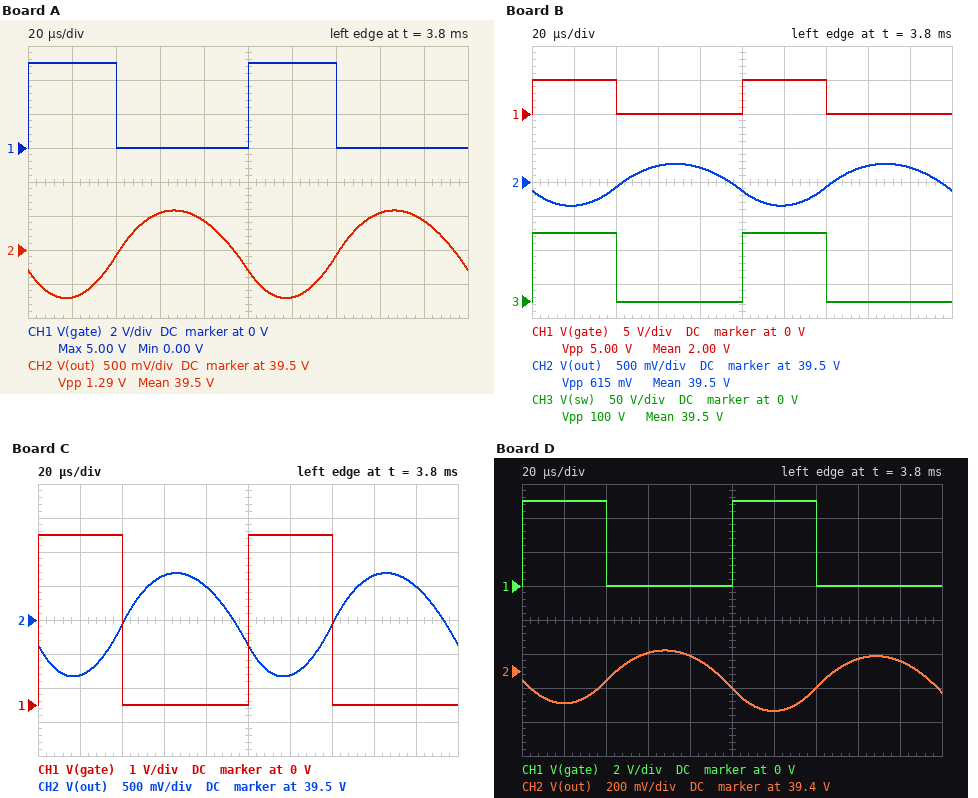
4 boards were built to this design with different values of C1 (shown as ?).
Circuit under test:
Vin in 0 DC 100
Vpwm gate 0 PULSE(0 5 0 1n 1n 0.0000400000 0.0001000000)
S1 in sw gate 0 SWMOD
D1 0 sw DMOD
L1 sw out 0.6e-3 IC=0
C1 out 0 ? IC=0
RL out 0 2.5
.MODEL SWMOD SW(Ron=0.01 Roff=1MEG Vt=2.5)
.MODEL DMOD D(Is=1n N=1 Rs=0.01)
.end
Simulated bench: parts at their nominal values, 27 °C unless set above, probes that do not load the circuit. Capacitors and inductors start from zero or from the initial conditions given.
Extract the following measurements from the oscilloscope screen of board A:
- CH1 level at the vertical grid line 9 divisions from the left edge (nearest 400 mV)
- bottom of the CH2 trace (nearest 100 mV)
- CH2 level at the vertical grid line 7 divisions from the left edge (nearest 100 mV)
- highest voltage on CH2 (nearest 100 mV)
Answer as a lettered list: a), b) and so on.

a) 0 V
b) 38.8 V
c) 39.4 V
d) 40.1 V
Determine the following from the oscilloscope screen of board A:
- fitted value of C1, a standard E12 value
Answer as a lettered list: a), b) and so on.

a) 39 µF
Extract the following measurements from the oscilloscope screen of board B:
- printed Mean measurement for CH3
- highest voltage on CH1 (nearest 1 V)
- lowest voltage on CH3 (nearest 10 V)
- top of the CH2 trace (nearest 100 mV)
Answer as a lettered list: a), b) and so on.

a) 39.5 V
b) 5 V
c) 0 V
d) 39.8 V
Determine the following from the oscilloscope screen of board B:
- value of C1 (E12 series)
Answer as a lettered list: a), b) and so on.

a) 82 µF
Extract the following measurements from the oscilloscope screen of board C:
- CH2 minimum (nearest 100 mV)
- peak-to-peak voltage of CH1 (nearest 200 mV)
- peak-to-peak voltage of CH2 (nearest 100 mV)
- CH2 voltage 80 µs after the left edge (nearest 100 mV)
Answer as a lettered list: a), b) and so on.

a) 38.7 V
b) 5.0 V
c) 1.5 V
d) 40.0 V
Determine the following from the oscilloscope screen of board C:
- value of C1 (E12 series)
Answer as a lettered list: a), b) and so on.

a) 33 µF
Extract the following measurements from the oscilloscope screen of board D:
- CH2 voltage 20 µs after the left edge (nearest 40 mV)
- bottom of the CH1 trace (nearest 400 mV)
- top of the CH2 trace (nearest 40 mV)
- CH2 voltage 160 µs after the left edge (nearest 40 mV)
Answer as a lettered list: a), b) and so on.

a) 39.20 V
b) 0 V
c) 39.52 V
d) 39.48 V
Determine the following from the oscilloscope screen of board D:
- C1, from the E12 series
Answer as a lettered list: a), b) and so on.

a) 150 µF
